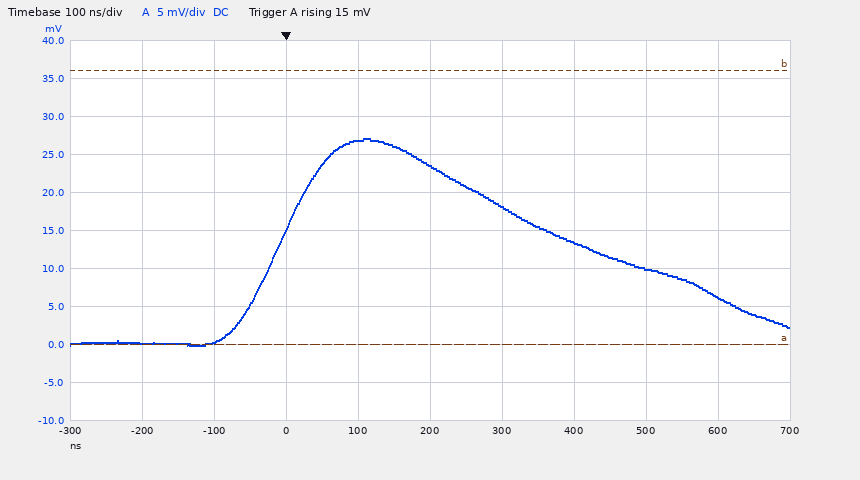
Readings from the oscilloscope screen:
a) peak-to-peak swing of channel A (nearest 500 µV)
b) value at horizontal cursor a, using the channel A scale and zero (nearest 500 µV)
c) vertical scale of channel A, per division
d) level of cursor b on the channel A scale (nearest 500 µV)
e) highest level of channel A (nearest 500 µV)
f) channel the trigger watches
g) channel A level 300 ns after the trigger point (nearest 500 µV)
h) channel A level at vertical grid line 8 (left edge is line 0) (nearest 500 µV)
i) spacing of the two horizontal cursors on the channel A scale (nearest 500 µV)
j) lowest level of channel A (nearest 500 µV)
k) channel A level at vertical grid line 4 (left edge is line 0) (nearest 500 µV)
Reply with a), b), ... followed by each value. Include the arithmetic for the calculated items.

a) 27.0 mV − (0.0 mV) = 27.0 mV
b) 0.0 mV
c) 5 mV
d) 36.0 mV
e) 27.0 mV
f) channel A
g) 18.0 mV
h) 10.0 mV
i) 36.0 mV
j) 0.0 mV
k) 27.0 mV
